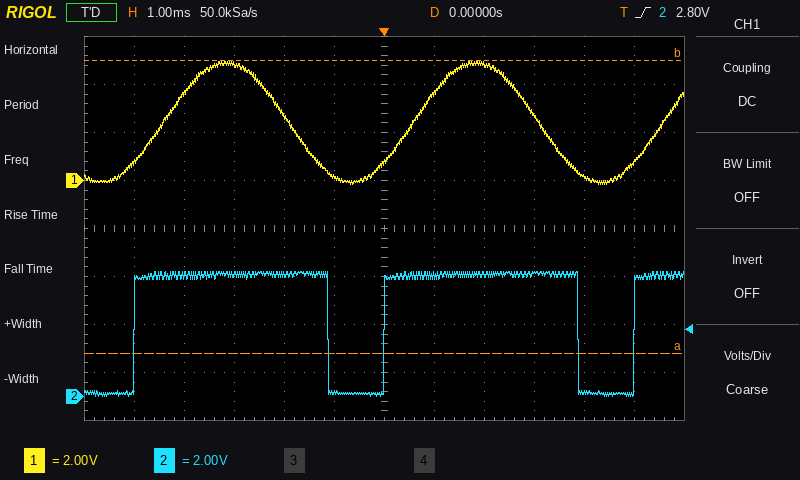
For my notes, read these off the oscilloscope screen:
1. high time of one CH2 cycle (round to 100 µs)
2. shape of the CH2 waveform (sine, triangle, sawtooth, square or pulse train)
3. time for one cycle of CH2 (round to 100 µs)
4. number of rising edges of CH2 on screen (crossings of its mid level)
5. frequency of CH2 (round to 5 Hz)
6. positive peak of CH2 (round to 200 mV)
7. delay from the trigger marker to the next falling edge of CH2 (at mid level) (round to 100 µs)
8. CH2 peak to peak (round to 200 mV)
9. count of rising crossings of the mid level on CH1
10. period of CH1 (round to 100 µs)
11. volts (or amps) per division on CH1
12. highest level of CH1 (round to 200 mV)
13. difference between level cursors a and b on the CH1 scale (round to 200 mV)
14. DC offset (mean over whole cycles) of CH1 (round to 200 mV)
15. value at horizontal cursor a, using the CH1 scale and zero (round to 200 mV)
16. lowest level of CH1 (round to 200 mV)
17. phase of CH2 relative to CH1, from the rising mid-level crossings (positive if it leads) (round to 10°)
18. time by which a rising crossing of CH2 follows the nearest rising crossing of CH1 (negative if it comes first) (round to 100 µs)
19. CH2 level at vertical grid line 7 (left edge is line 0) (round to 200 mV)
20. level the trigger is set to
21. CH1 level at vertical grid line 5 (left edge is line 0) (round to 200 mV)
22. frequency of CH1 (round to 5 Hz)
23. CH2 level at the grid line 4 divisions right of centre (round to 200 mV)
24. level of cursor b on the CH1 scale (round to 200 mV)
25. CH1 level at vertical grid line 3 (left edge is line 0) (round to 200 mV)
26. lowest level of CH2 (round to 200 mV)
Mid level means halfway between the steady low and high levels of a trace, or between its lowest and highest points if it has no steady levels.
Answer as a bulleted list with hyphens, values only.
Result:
- 3.9 ms
- pulse train
- 5.0 ms
- 3
- 200 Hz
- 5.2 V
- 3.9 ms
- 5.2 V
- 3
- 5.0 ms
- 2 V
- 5.0 V
- 12.2 V
- 2.4 V
- -7.2 V
- -200 mV
- +40°
- -600 µs
- 5.0 V
- 2.80 V
- 200 mV
- 200 Hz
- 200 mV
- 5.0 V
- 4.8 V
- 0.0 V
